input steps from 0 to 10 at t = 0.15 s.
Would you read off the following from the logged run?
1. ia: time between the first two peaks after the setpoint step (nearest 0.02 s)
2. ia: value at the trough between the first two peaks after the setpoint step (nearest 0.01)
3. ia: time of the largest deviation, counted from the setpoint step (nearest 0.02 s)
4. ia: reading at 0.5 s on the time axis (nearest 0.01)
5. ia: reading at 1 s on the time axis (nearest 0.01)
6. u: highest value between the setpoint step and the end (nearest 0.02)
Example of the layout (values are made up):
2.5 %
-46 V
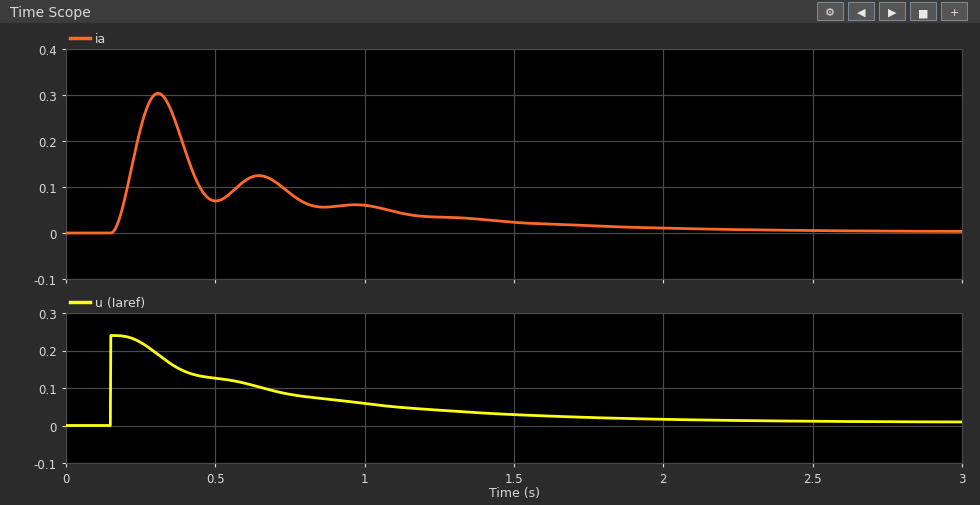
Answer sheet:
0.34 s
0.07
0.16 s
0.07
0.06
0.24
